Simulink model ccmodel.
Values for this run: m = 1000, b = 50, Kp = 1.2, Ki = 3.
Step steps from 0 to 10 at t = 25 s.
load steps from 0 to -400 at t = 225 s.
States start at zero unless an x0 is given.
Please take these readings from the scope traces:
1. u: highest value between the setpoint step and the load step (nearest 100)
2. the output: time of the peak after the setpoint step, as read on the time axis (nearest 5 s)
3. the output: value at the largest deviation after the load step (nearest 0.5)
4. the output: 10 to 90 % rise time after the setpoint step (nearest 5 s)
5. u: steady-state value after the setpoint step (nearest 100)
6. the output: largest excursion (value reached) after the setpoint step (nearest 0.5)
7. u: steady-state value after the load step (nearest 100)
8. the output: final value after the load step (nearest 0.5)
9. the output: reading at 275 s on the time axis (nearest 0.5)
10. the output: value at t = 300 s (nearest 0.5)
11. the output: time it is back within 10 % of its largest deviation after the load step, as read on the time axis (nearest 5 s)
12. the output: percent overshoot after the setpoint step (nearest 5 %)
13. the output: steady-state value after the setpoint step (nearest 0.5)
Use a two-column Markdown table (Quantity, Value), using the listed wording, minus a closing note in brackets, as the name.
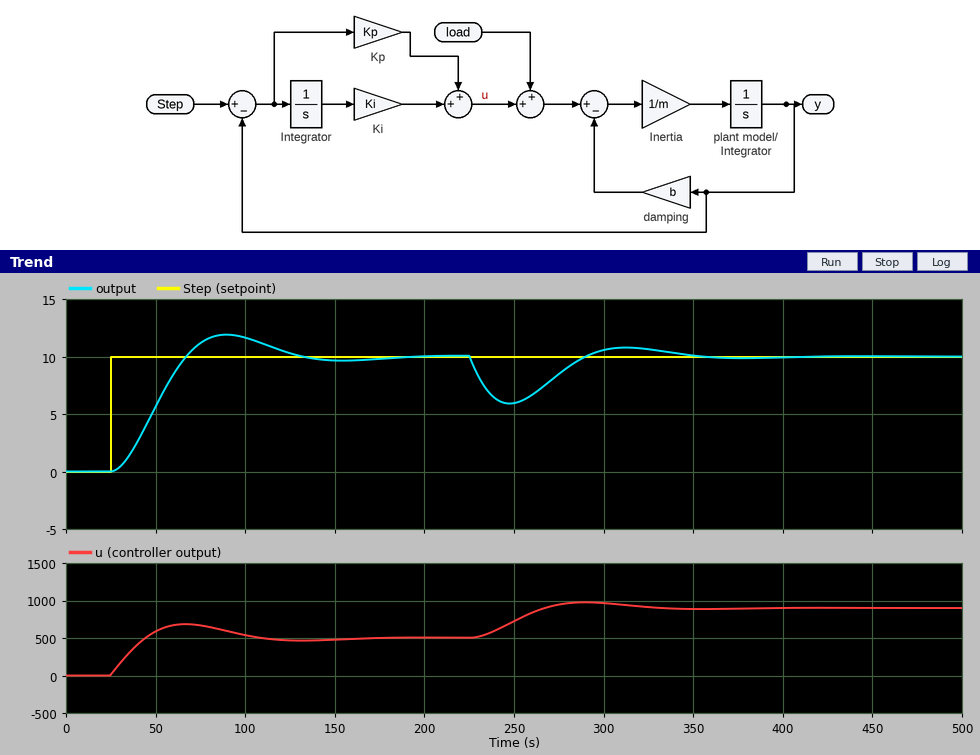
| Quantity | Value |
|---|---|
| u: highest value between the setpoint step and the load step | 700 |
| the output: time of the peak after the setpoint step, as read on the time axis | 90 s |
| the output: value at the largest deviation after the load step | 6.0 |
| the output: 10 to 90 % rise time after the setpoint step | 30 s |
| u: steady-state value after the setpoint step | 500 |
| the output: largest excursion (value reached) after the setpoint step | 12.0 |
| u: steady-state value after the load step | 900 |
| the output: final value after the load step | 10.0 |
| the output: reading at 275 s on the time axis | 8.5 |
| the output: value at t = 300 s | 10.5 |
| the output: time it is back within 10 % of its largest deviation after the load step, as read on the time axis | 335 s |
| the output: percent overshoot after the setpoint step | 20 % |
| the output: steady-state value after the setpoint step | 10.0 |
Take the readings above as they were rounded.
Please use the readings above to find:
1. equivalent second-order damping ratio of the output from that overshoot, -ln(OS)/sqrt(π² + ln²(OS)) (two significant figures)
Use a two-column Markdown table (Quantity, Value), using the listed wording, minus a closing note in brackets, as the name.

| Quantity | Value |
|---|---|
| equivalent second-order damping ratio of the output from that overshoot, -ln(OS)/sqrt(π² + ln²(OS)) | 0.46 |
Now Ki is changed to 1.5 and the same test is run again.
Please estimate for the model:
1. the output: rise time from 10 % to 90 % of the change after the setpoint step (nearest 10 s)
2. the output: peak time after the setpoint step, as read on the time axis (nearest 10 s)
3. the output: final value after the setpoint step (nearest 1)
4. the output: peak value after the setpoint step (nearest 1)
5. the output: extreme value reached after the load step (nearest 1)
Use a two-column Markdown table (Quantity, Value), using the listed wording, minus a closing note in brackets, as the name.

| Quantity | Value |
|---|---|
| the output: rise time from 10 % to 90 % of the change after the setpoint step | 50 s |
| the output: peak time after the setpoint step, as read on the time axis | 130 s |
| the output: final value after the setpoint step | 10 |
| the output: peak value after the setpoint step | 11 |
| the output: extreme value reached after the load step | 5 |
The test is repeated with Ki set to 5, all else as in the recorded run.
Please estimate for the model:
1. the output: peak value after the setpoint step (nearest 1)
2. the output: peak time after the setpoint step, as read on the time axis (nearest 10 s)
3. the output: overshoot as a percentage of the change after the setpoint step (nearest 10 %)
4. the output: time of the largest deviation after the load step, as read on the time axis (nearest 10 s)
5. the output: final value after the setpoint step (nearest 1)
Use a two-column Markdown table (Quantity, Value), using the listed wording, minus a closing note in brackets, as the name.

| Quantity | Value |
|---|---|
| the output: peak value after the setpoint step | 13 |
| the output: peak time after the setpoint step, as read on the time axis | 70 s |
| the output: overshoot as a percentage of the change after the setpoint step | 30 % |
| the output: time of the largest deviation after the load step, as read on the time axis | 240 s |
| the output: final value after the setpoint step | 10 |
